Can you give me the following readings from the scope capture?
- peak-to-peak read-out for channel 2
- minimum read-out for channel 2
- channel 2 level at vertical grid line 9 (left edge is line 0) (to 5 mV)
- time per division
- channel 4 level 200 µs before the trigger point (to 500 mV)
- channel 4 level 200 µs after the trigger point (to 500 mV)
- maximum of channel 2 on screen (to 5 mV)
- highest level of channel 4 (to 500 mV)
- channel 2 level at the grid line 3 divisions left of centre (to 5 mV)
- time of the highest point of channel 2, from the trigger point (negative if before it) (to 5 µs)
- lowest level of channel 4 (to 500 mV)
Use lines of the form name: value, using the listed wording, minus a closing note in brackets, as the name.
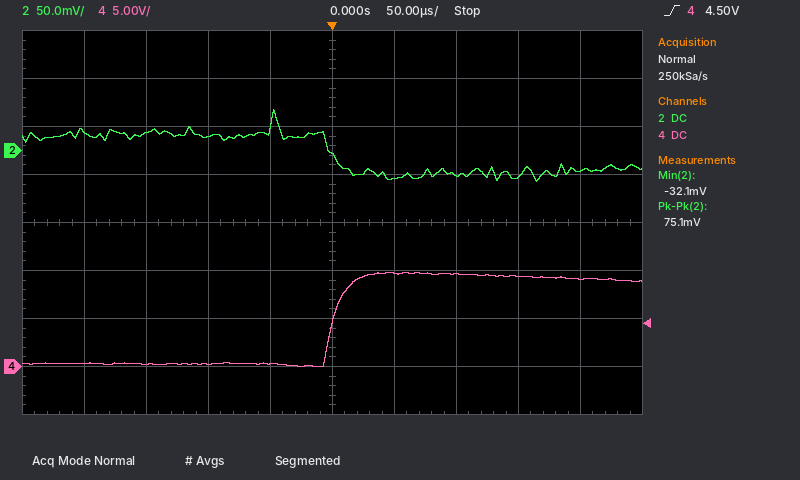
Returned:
peak-to-peak read-out for channel 2: 75.1 mV
minimum read-out for channel 2: -32.1 mV
channel 2 level at vertical grid line 9 (left edge is line 0): -20 mV
time per division: 50 µs
channel 4 level 200 µs before the trigger point: 500 mV
channel 4 level 200 µs after the trigger point: 9.0 V
maximum of channel 2 on screen: 45 mV
highest level of channel 4: 10.0 V
channel 2 level at the grid line 3 divisions left of centre: 20 mV
time of the highest point of channel 2, from the trigger point (negative if before it): -45 µs
lowest level of channel 4: 0.0 V
